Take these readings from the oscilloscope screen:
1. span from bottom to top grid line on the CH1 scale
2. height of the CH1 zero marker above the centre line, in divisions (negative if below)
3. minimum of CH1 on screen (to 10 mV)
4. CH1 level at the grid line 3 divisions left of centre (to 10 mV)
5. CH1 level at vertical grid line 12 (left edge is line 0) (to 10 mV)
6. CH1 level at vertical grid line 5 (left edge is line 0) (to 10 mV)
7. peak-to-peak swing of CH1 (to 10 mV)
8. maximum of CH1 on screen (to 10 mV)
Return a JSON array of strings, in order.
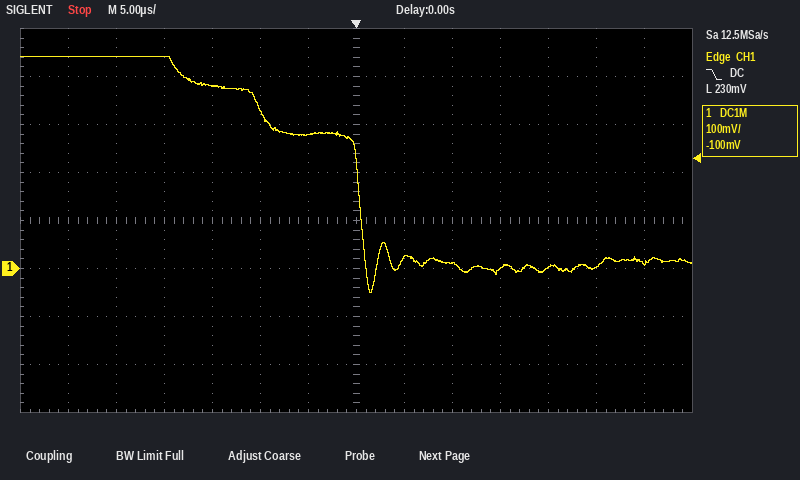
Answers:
["800 mV", "-1.0 div", "-50 mV", "380 mV", "0 mV", "330 mV", "490 mV", "440 mV"]
